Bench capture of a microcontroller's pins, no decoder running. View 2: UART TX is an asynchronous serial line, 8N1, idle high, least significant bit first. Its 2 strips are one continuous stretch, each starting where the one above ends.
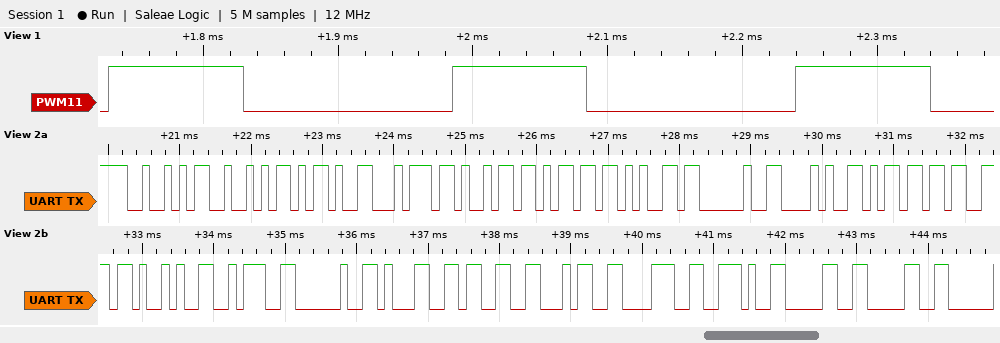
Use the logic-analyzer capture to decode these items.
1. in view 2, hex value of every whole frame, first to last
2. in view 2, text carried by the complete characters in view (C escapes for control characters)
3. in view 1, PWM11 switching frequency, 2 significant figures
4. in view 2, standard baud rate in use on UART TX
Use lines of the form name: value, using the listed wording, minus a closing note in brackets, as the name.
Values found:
in view 2, hex value of every whole frame, first to last: 52 52 2D 74 69 6D 65 20 28 6D 73 29 3A 20 31 33 34 38 2E 30 30
in view 2, text carried by the complete characters in view: "RR-time (ms): 1348.00"
in view 1, PWM11 switching frequency, 2 significant figures: 3.9 kHz
in view 2, standard baud rate in use on UART TX: 9600 baud
